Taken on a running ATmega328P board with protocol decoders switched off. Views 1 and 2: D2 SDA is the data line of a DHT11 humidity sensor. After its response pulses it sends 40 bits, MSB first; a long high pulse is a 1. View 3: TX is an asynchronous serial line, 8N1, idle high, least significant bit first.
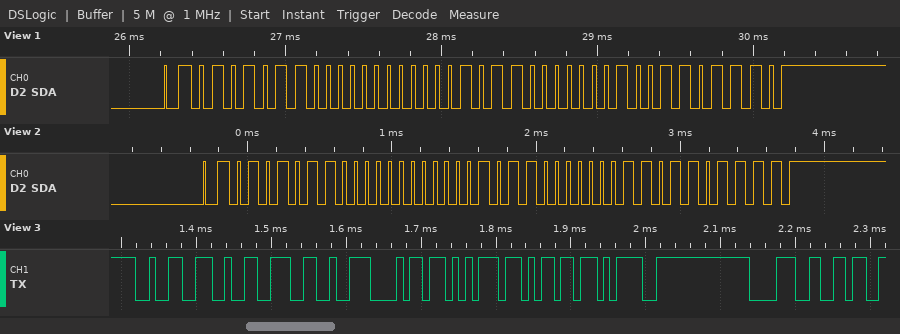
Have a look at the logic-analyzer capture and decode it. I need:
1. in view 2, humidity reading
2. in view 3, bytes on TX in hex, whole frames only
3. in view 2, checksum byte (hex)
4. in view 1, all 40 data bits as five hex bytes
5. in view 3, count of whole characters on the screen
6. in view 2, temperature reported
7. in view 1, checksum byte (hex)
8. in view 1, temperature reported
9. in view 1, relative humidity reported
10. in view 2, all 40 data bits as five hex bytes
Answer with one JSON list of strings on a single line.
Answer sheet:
["86 %", "0x32 0x32 0x26 0x68 0x75 0x6D 0x3D 0x38 0x36", "0x6F", "56 00 16 02 6E", "9", "22.3 °C", "0x6E", "22.2 °C", "86 %", "56 00 16 03 6F"]
